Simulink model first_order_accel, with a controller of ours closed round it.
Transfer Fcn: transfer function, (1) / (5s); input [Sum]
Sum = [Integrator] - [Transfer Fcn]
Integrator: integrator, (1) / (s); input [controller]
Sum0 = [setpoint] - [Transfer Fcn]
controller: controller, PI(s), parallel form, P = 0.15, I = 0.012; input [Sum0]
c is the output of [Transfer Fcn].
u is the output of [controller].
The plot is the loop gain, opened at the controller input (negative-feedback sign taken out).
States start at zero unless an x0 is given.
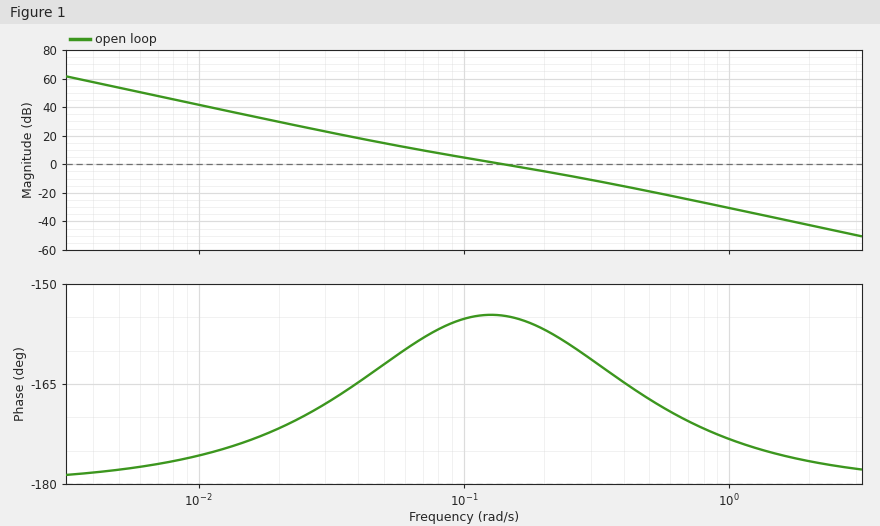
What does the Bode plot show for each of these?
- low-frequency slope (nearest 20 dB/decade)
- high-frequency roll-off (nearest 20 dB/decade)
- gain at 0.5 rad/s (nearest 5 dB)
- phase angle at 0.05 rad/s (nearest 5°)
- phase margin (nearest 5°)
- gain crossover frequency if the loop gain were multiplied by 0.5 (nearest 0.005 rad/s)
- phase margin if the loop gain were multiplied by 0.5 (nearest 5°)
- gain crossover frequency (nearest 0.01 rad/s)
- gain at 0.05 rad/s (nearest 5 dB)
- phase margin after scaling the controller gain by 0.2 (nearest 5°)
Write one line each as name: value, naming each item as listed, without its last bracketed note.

low-frequency slope: -40 dB/decade
high-frequency roll-off: -40 dB/decade
gain at 0.5 rad/s: -20 dB
phase angle at 0.05 rad/s: -160°
phase margin: 25°
gain crossover frequency if the loop gain were multiplied by 0.5: 0.090 rad/s
phase margin if the loop gain were multiplied by 0.5: 25°
gain crossover frequency: 0.14 rad/s
gain at 0.05 rad/s: 15 dB
phase margin after scaling the controller gain by 0.2: 20°
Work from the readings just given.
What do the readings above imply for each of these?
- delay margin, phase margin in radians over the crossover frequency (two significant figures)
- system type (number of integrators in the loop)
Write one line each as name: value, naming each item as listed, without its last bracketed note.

delay margin, phase margin in radians over the crossover frequency: 3.1 s
system type: 2
